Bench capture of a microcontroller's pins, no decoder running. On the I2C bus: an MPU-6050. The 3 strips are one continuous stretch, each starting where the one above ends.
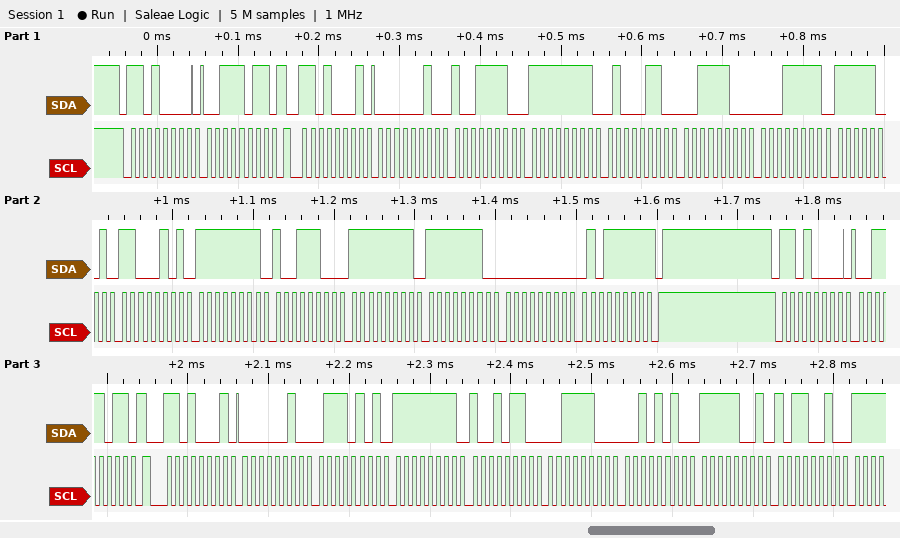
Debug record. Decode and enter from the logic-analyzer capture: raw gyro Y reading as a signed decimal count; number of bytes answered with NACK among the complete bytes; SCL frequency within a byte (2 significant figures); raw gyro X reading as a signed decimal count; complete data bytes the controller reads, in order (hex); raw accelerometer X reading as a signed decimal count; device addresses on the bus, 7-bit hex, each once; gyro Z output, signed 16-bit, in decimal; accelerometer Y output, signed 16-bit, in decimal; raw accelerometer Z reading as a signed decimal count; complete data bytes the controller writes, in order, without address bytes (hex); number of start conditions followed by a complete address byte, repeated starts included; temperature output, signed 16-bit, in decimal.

-2
1
100 kHz
-100
02 9E FF 46 3C 1F F9 C5 FF 9C FF FE 00 5F 02 75 FF 96 3C 2A F9 B2
670
0x68
95
-186
15391
3B 3B
4
-1595
